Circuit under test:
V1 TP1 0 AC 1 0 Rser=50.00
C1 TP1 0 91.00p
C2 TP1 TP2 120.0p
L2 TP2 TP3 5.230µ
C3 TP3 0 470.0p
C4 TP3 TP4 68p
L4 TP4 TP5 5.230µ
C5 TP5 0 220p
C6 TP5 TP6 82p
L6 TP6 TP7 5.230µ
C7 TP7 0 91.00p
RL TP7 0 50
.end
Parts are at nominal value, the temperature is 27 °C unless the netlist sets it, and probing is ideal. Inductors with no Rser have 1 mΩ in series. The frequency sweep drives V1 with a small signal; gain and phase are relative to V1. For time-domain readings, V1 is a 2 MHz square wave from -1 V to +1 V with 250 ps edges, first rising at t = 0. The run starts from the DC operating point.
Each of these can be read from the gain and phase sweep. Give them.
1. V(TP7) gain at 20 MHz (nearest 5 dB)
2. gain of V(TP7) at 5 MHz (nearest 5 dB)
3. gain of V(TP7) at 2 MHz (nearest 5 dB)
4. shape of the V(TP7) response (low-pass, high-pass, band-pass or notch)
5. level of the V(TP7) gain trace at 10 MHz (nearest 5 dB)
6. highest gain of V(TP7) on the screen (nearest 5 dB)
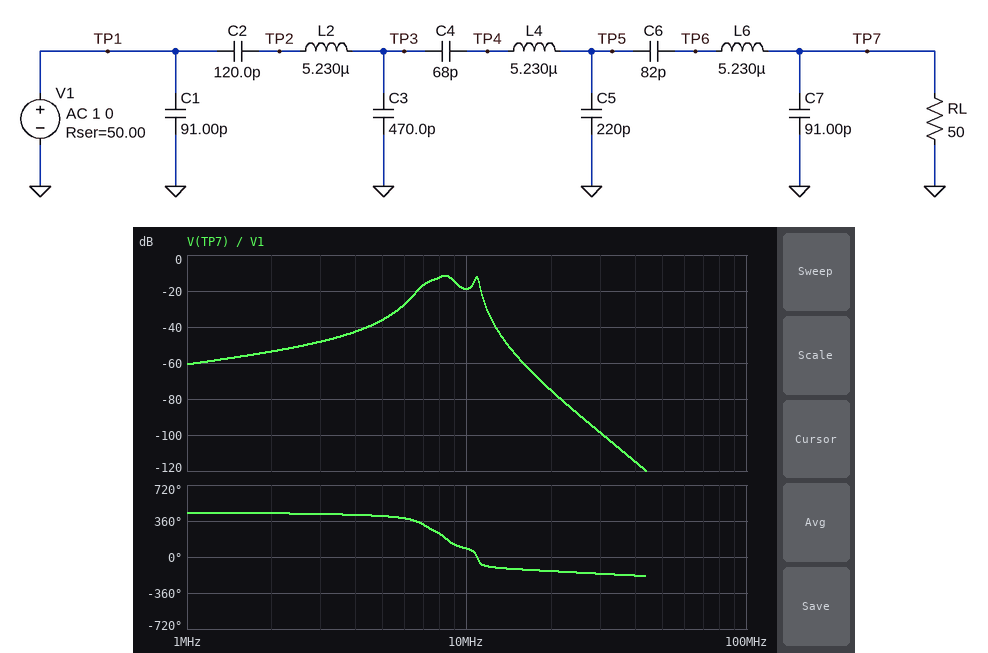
-75 dB
-35 dB
-55 dB
band-pass
-20 dB
-10 dB
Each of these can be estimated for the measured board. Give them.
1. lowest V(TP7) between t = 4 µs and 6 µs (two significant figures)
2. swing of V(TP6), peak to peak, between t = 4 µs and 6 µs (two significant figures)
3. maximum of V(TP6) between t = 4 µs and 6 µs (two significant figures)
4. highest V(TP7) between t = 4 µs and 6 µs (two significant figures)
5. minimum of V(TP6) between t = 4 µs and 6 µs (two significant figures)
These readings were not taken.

-46 mV
520 mV
260 mV
46 mV
-260 mV
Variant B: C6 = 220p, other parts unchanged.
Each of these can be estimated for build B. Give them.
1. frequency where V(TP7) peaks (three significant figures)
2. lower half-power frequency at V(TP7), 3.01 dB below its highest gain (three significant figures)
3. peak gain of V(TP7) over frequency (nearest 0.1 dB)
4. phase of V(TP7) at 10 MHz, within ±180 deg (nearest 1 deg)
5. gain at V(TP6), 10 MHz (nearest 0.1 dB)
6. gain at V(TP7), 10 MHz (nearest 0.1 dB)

10.6 MHz
10.5 MHz
-7.8 dB
79 deg
-5.0 dB
-21.4 dB
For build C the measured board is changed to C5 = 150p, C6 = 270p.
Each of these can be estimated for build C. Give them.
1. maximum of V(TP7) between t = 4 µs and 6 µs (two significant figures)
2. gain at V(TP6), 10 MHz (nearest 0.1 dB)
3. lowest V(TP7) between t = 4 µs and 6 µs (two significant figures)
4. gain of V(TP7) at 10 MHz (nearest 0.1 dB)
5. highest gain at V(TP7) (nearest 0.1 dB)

110 mV
-8.8 dB
-110 mV
-25.2 dB
-10.7 dB
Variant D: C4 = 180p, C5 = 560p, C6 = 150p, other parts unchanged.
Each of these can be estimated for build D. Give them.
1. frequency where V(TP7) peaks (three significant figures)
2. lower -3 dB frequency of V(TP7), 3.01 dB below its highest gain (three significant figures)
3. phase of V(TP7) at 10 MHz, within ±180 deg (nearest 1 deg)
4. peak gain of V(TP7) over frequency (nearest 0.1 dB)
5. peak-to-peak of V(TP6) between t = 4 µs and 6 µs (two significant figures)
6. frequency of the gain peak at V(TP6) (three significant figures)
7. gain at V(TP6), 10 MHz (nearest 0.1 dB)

6.72 MHz
5.65 MHz
-89 deg
-6.2 dB
1.6 V
6.86 MHz
-24.3 dB
